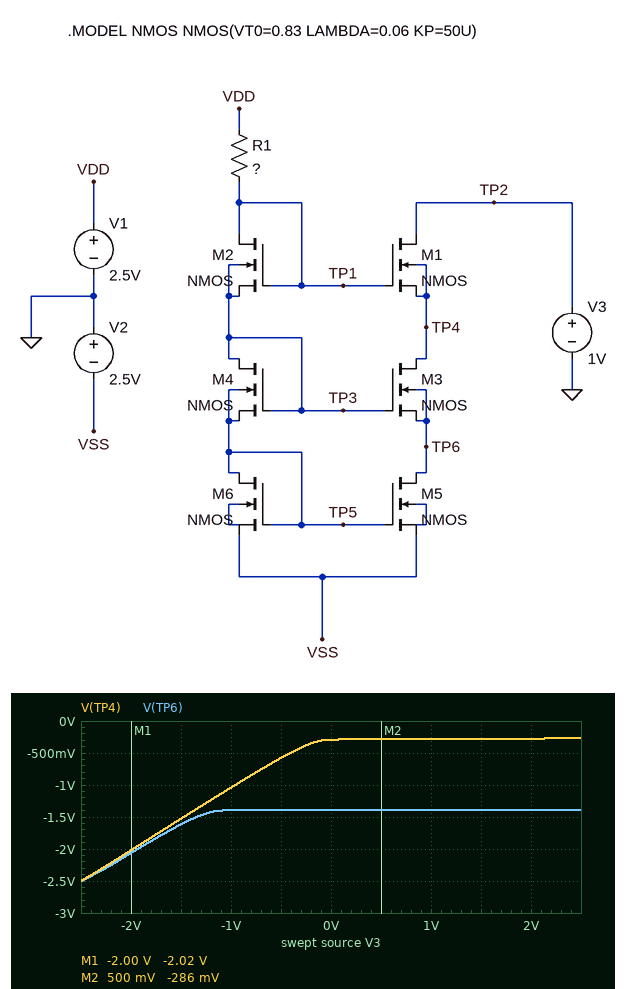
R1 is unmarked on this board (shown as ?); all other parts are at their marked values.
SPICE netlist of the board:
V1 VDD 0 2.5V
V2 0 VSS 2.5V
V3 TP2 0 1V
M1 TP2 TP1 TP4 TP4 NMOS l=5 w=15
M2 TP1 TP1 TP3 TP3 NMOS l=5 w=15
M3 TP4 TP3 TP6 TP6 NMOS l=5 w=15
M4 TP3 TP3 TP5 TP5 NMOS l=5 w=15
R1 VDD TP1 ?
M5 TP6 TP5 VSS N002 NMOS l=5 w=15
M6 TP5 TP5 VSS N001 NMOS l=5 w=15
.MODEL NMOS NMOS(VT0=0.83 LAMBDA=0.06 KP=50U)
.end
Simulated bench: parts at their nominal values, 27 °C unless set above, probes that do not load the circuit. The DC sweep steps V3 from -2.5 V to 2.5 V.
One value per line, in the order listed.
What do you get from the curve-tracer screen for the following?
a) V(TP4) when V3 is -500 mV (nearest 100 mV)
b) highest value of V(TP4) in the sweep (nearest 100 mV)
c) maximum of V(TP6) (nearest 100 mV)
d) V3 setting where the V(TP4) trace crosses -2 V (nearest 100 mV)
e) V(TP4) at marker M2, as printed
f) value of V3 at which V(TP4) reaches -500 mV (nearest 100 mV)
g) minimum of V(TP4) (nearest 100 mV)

-600 mV
-300 mV
-1.4 V
-2.0 V
-286 mV
-400 mV
-2.5 V
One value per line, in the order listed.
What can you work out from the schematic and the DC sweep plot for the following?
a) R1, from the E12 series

270 kΩ
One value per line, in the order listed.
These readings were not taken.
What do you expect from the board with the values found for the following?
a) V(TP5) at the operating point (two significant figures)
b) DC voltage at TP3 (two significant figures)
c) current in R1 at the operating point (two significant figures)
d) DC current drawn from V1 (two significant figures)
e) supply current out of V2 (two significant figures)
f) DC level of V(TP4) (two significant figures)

-1.4 V
-280 mV
6.2 µA
6.2 µA
12 µA
-280 mV
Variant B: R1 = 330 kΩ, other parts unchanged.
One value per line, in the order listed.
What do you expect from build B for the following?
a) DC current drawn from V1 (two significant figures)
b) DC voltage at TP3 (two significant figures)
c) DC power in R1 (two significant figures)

5.3 µA
-330 mV
9.2 µW
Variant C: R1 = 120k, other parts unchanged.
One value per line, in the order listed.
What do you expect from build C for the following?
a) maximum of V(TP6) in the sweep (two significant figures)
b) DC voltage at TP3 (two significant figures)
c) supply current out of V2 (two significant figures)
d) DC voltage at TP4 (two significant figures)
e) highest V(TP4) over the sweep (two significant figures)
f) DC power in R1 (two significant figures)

-1.3 V
-85 mV
23 µA
-86 mV
-71 mV
16 µW
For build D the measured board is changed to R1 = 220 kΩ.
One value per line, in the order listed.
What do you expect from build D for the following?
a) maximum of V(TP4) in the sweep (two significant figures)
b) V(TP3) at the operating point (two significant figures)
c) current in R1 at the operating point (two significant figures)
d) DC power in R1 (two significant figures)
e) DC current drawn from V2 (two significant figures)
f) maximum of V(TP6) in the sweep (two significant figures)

-220 mV
-240 mV
7.3 µA
12 µW
15 µA
-1.4 V
